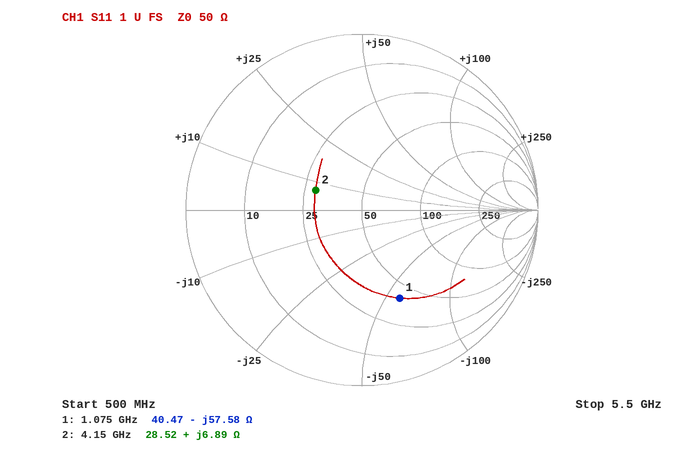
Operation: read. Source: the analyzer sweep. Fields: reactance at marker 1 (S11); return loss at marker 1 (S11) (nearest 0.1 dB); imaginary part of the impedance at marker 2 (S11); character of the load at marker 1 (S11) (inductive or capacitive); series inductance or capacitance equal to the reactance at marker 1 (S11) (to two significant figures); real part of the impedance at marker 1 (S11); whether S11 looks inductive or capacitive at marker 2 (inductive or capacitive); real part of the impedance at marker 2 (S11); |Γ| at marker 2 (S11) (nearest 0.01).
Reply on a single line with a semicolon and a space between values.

-57.58 Ω; 5.3 dB; +6.89 Ω; capacitive; 2.6 pF; 40.47 Ω; inductive; 28.52 Ω; 0.29
